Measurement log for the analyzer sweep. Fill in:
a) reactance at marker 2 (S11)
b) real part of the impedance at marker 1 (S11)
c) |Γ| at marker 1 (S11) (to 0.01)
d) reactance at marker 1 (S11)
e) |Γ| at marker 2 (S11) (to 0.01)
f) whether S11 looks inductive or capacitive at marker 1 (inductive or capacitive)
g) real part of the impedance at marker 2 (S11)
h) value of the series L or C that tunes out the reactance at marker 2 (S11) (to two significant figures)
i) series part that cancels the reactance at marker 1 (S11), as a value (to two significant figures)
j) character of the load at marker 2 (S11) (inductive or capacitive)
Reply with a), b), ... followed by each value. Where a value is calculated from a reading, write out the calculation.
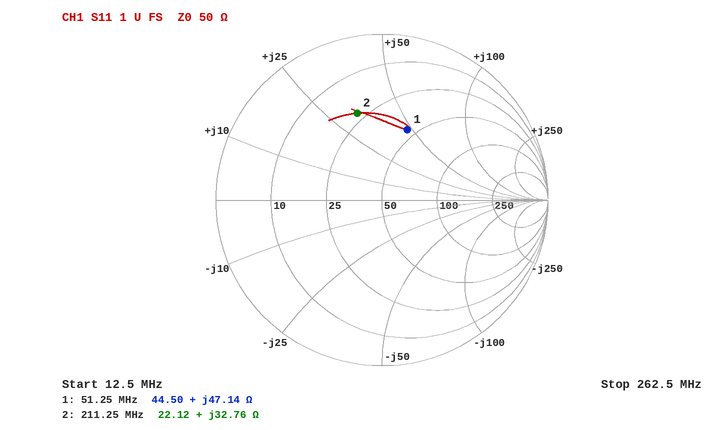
a) +32.76 Ω
b) 44.50 Ω
c) 0.45
d) +47.14 Ω
e) 0.54
f) inductive
g) 22.12 Ω
h) C = 1/(2π × 211.25 MHz × 32.76 Ω) ≈ 23 pF
i) C = 1/(2π × 51.25 MHz × 47.14 Ω) ≈ 66 pF
j) inductive
